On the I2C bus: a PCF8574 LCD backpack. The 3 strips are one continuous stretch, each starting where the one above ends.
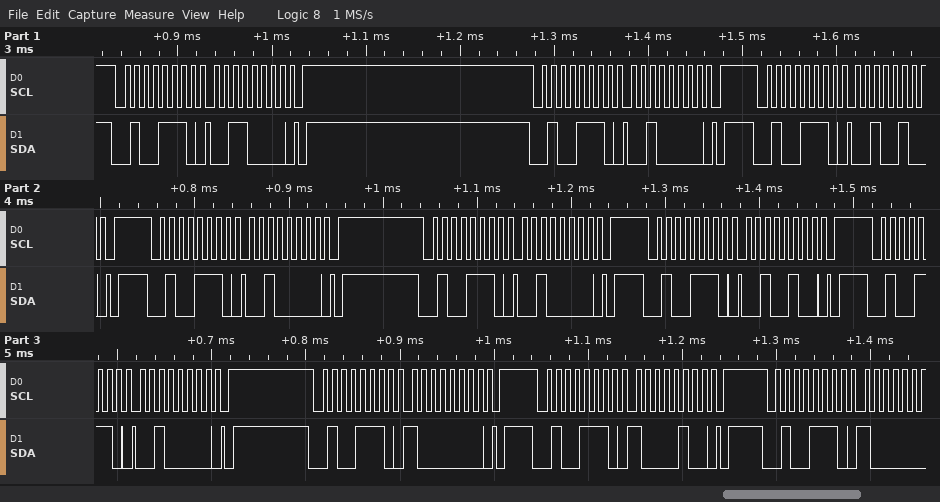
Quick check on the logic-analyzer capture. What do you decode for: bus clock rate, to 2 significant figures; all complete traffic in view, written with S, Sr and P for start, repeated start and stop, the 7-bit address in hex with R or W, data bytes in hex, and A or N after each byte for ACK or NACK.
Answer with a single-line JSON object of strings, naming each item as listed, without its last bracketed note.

{"bus clock rate, to 2 significant figures": "100 kHz", "all complete traffic in view, written with S, Sr and P for start, repeated start and stop, the 7-bit address in hex with R or W, data bytes in hex, and A or N after each byte for ACK or NACK": "S 27W A 30 A P S 27W A 20 A P S 27W A 24 A P S 27W A 20 A P S 27W A 20 A P S 27W A 24 A P S 27W A 20 A P S 27W A 80 A P S 27W A 84 A P S 27W A"}
